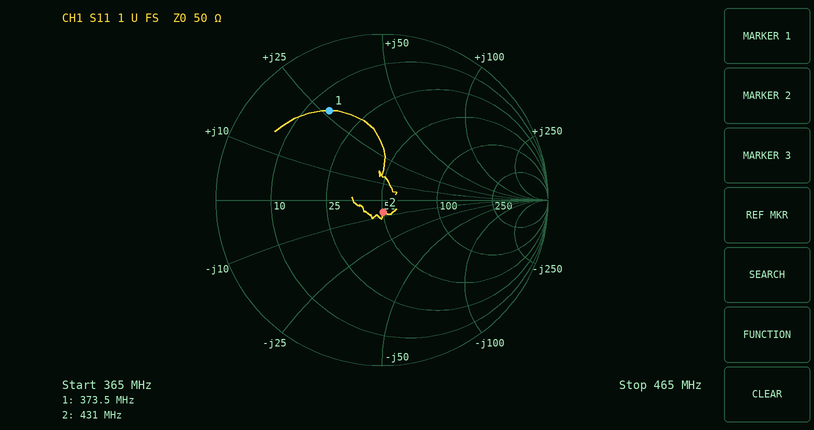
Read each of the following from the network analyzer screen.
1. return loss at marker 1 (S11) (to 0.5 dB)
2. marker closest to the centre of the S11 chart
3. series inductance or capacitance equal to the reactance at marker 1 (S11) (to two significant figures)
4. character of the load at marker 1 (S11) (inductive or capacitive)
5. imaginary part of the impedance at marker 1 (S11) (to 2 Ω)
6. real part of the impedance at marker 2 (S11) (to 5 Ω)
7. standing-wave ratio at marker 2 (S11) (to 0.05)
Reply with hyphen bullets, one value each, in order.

- 4.0 dB
- marker 2
- 11 nH
- inductive
- +26 Ω
- 50 Ω
- 1.15
